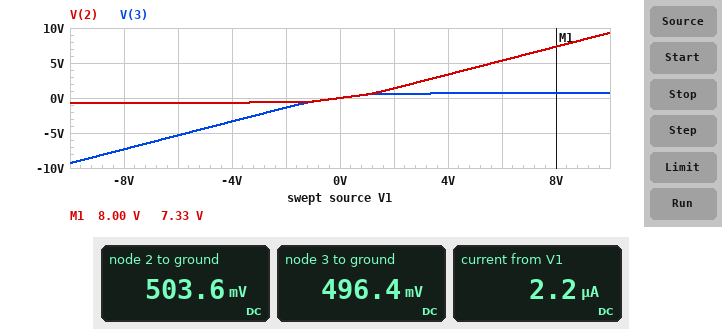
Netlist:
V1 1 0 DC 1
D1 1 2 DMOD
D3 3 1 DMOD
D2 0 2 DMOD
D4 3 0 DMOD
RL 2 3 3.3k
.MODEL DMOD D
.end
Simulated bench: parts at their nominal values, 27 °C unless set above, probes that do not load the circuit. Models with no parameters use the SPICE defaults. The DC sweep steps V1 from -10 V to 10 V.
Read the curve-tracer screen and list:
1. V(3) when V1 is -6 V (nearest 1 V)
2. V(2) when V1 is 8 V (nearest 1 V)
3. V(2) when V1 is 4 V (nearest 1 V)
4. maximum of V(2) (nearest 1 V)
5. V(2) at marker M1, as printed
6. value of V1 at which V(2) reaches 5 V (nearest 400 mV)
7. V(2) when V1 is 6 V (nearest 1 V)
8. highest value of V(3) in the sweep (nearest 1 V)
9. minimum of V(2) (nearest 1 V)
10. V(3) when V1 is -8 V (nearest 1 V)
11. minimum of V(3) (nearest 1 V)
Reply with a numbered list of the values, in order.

1. -5 V
2. 7 V
3. 3 V
4. 9 V
5. 7.33 V
6. 5.6 V
7. 5 V
8. 1 V
9. -1 V
10. -7 V
11. -9 V
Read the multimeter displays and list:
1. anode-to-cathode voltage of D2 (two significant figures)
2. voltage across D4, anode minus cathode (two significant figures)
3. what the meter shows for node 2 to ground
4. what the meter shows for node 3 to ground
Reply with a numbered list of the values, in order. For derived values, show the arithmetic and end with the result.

1. 0 V - 503.6 mV = -500 mV
2. 496.4 mV = 500 mV
3. 503.6 mV
4. 496.4 mV
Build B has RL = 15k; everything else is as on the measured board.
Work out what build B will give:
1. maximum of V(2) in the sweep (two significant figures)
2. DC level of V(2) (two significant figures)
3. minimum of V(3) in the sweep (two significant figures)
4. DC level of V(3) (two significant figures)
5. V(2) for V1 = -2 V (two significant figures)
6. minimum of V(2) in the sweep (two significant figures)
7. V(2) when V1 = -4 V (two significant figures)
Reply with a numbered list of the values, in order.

1. 9.4 V
2. 510 mV
3. -9.4 V
4. 490 mV
5. -580 mV
6. -640 mV
7. -610 mV
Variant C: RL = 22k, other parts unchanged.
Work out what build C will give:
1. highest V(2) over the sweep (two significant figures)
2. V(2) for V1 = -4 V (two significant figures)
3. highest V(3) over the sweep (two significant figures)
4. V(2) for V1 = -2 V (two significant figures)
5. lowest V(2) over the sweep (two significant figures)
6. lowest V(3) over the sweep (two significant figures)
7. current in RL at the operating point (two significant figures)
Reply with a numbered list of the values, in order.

1. 9.4 V
2. -600 mV
3. 630 mV
4. -570 mV
5. -630 mV
6. -9.4 V
7. 1.4 µA
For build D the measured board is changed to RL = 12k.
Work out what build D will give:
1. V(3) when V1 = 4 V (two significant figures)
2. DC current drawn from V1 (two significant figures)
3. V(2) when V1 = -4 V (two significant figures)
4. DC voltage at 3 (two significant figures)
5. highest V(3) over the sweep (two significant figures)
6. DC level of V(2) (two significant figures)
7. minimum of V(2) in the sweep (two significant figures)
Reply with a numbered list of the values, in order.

1. 620 mV
2. 1.7 µA
3. -620 mV
4. 490 mV
5. 650 mV
6. 510 mV
7. -650 mV
